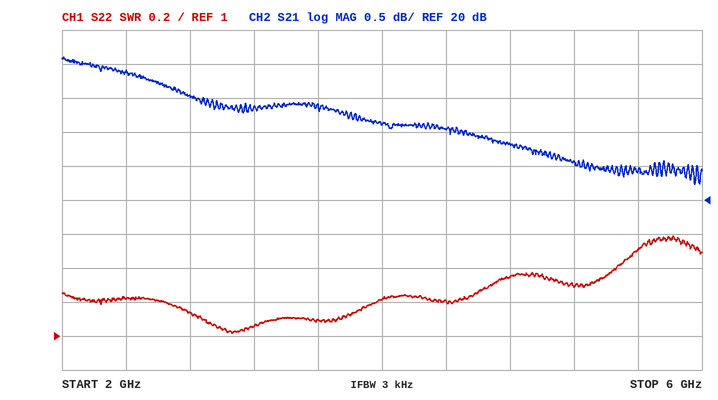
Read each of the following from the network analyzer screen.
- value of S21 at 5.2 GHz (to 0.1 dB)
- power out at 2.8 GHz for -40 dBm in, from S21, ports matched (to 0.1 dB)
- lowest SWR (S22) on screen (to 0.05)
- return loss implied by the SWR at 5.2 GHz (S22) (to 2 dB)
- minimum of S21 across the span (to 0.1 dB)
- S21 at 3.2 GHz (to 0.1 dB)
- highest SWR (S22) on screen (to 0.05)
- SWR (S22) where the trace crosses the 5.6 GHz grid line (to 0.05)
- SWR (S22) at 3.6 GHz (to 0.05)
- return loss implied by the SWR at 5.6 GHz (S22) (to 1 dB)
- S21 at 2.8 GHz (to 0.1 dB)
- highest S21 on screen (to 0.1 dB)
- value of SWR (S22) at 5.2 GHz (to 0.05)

20.6 dB
-18.5 dBm
1.00
18 dB
20.2 dB
21.4 dB
1.60
1.50
1.10
14 dB
21.5 dB
22.1 dB
1.30
